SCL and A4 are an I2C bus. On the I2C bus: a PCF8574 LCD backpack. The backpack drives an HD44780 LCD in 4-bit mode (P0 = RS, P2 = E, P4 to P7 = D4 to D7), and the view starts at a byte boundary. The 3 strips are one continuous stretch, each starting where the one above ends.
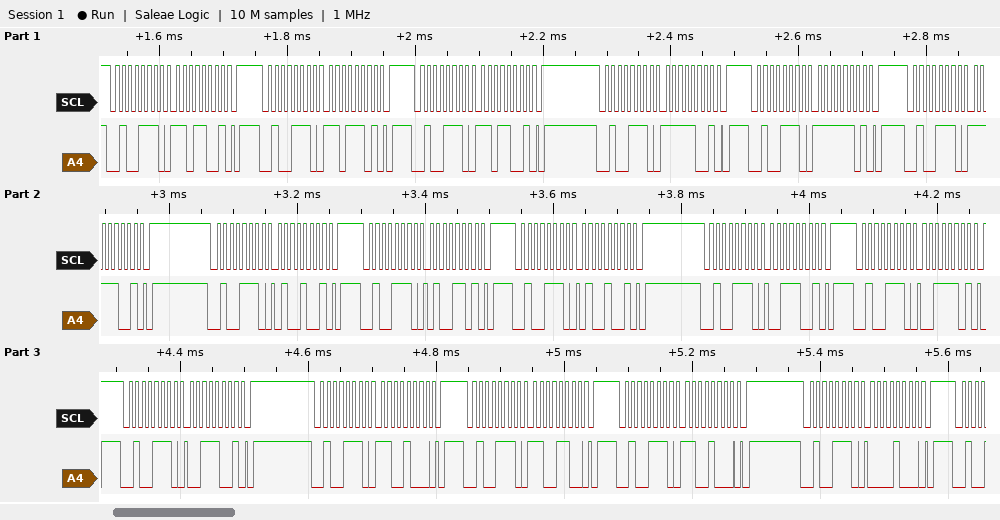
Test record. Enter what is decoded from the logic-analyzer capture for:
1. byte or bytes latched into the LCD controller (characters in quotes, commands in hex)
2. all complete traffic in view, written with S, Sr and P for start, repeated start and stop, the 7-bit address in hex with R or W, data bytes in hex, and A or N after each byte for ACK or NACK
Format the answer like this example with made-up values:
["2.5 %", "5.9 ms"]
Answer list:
["data 0xDF 'C'", "S 27W A D9 A P S 27W A DD A P S 27W A D9 A P S 27W A F9 A P S 27W A FD A P S 27W A F9 A P S 27W A 49 A P S 27W A 4D A P S 27W A 49 A P S 27W A 39 A P S 27W A 3D A P S 27W A 39 A P S 27W A C8 A P S 27W A CC A P S 27W A C8 A P S 27W A 08 A P"]
